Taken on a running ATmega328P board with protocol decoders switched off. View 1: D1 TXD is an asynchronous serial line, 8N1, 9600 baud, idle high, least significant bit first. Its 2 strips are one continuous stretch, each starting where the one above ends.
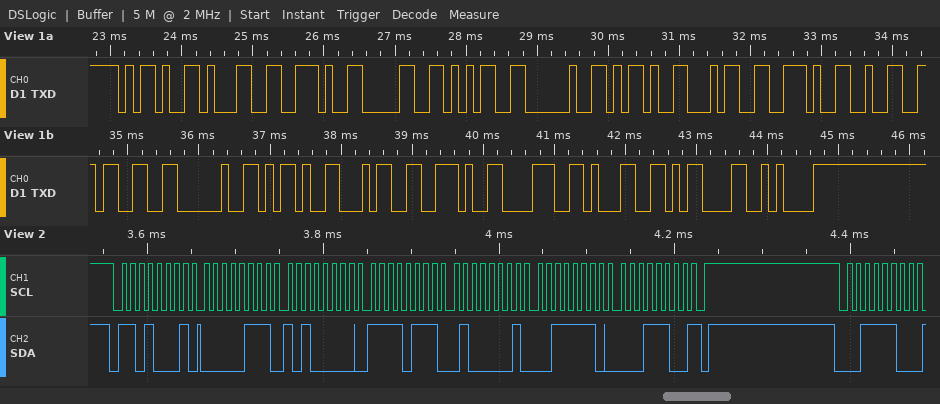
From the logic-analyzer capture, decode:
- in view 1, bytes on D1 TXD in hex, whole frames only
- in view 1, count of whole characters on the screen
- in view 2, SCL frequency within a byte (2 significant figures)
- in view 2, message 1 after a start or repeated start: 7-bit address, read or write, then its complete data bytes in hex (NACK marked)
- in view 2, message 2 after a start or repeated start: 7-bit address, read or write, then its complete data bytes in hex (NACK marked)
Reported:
2D 31 2E 30 35 20 2D 34 2E 32 33 20 2D 34 2E 38 31 0D 0A
19
100 kHz
0x68 read: 07 A0 F7 41 3E 1C NACK
0x1E write
